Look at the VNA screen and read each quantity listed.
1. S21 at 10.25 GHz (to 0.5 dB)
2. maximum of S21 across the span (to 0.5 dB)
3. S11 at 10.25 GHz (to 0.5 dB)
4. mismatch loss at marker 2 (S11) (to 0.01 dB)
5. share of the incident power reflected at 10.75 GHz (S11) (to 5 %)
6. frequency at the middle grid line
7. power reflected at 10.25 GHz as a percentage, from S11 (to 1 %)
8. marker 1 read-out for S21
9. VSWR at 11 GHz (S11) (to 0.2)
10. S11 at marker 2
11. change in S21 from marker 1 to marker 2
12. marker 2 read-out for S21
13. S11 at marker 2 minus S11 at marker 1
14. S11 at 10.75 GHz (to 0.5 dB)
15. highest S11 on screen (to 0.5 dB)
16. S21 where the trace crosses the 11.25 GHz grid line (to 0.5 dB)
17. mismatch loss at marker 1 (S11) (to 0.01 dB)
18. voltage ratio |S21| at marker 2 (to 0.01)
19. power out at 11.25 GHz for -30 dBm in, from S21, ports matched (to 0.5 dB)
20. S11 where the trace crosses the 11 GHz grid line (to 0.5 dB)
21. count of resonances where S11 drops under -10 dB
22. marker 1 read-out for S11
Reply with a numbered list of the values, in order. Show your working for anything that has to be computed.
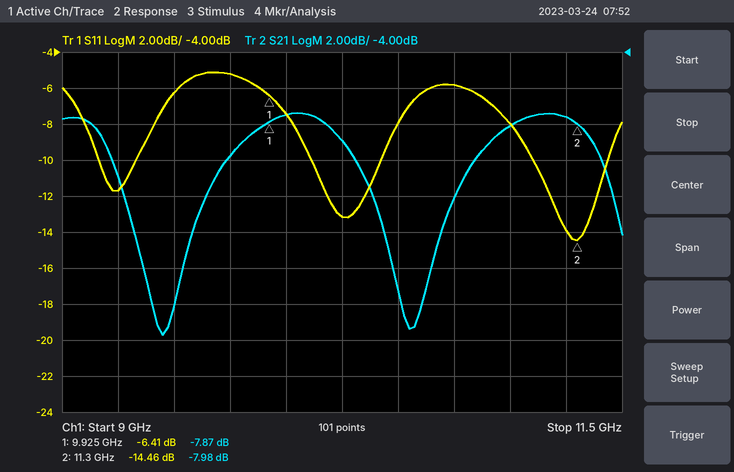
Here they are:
1. -9.0 dB
2. -7.5 dB
3. -13.0 dB
4. −10 log10(1 − 10^(-14.46/10)) ≈ 0.16 dB
5. 10^(-6/10) ≈ 25 %
6. 10.25 GHz
7. 10^(-13/10) ≈ 5 %
8. -7.87 dB
9. |Γ| = 10^(-8/20) = 0.3981; VSWR = (1 + 0.3981)/(1 − 0.3981) ≈ 2.32, so 2.4 to the nearest 0.2
10. -14.46 dB
11. -7.98 − (-7.87) = -0.11 dB
12. -7.98 dB
13. -14.46 − (-6.41) = -8.05 dB
14. -6.0 dB
15. -5.0 dB
16. -7.5 dB
17. −10 log10(1 − 10^(-6.41/10)) ≈ 1.13 dB
18. 10^(-7.98/20) ≈ 0.40
19. -30 dBm + (-7.5 dB) = -37.5 dBm
20. -8.0 dB
21. 3
22. -6.41 dB
